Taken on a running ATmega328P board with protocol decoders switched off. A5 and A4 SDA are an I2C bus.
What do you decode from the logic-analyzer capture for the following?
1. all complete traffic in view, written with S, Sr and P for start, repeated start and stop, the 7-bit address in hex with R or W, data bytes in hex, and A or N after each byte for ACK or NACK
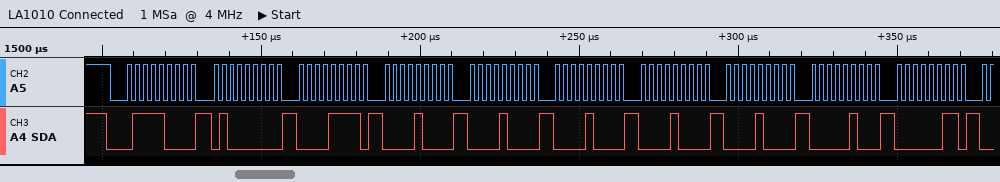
S 3CW A 40 A 0F A 08 A 08 A 08 A 08 A 08 A 04 A 03 A
